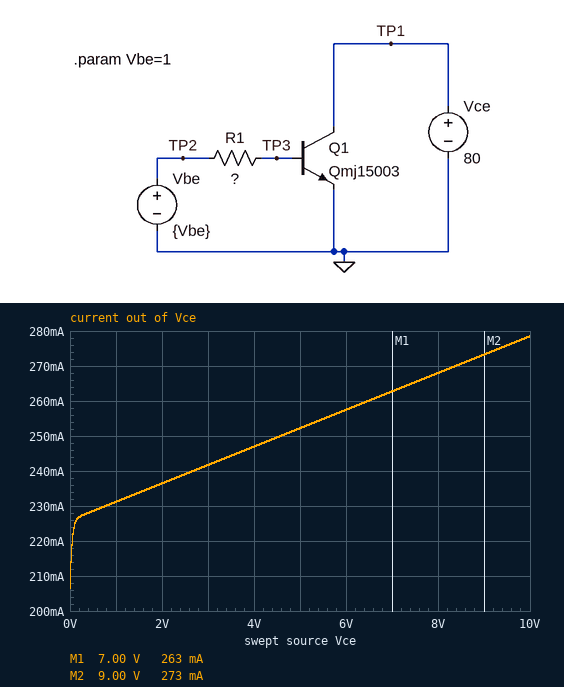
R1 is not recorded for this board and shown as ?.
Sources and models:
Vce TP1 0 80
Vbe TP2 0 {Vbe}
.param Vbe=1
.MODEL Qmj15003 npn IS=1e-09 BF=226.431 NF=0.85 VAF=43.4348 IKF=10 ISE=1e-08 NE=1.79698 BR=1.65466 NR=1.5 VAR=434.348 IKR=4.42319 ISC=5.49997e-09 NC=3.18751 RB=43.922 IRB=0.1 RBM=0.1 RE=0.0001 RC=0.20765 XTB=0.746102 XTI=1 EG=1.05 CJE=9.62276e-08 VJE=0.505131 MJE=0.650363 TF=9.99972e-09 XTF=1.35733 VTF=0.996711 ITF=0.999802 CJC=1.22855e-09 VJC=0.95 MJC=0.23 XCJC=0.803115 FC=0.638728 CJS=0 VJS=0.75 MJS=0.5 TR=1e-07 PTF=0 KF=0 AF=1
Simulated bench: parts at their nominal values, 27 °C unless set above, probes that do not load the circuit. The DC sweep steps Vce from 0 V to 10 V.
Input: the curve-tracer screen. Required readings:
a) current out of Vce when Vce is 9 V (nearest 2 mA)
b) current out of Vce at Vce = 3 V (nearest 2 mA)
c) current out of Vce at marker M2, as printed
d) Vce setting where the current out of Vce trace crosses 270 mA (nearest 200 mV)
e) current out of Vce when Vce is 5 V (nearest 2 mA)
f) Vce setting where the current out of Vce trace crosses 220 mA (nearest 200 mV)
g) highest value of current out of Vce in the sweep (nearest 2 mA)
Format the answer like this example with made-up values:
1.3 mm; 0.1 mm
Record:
274 mA; 242 mA; 273 mA; 8.4 V; 252 mA; 0 V; 278 mA
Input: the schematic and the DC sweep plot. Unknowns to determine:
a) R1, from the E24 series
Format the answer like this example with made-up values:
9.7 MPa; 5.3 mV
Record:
470 Ω
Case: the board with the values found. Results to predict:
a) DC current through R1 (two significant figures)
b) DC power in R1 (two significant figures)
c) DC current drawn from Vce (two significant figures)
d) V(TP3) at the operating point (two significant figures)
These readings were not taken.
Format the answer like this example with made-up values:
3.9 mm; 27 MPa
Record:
1.1 mA; 590 µW; 650 mA; 470 mV
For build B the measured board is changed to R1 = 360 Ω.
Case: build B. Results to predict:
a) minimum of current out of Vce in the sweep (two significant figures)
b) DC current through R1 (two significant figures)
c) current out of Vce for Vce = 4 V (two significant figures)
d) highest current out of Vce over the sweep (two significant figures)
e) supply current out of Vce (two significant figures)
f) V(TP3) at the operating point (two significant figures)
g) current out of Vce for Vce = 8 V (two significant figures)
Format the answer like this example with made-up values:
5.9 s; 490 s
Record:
260 mA; 1.4 mA; 310 mA; 350 mA; 820 mA; 490 mV; 340 mA
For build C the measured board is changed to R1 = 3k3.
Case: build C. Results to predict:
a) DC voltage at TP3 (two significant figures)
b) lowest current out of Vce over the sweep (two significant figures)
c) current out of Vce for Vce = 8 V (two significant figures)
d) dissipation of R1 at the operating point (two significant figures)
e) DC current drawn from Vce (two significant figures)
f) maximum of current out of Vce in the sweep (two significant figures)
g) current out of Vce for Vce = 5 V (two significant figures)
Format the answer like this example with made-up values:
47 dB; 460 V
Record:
390 mV; 31 mA; 39 mA; 110 µW; 95 mA; 41 mA; 37 mA
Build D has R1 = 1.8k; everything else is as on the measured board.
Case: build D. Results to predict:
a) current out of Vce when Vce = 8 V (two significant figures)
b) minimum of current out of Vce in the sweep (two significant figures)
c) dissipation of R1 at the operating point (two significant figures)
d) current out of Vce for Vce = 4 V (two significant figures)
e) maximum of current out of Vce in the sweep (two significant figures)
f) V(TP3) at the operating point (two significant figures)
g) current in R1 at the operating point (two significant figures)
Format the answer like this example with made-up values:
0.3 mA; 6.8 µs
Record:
74 mA; 58 mA; 190 µW; 68 mA; 77 mA; 410 mV; 330 µA
